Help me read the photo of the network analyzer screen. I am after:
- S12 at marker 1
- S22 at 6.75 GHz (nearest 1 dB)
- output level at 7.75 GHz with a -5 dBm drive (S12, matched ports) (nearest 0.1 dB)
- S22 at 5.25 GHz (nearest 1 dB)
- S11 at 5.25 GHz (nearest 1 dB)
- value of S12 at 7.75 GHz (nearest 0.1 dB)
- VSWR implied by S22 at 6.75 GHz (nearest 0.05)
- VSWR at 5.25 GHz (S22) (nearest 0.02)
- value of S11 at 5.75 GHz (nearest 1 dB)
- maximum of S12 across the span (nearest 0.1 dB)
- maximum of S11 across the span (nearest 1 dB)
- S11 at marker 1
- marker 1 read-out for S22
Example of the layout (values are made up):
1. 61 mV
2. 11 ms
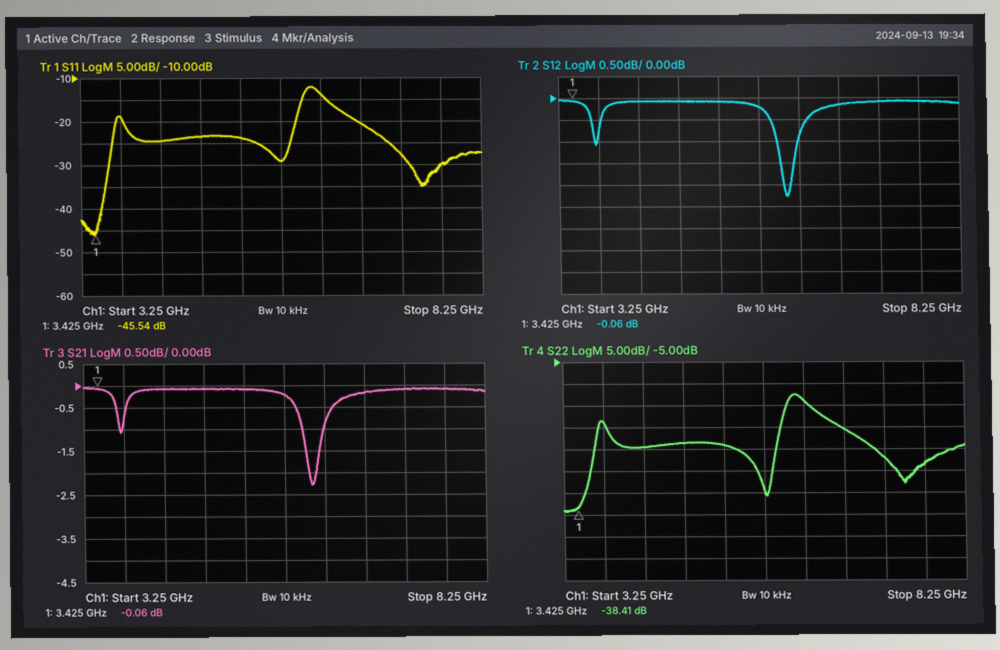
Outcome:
1. -0.06 dB
2. -20 dB
3. -5.1 dBm
4. -24 dB
5. -24 dB
6. -0.1 dB
7. 1.20
8. 1.14
9. -29 dB
10. 0.0 dB
11. -12 dB
12. -45.54 dB
13. -38.41 dB
